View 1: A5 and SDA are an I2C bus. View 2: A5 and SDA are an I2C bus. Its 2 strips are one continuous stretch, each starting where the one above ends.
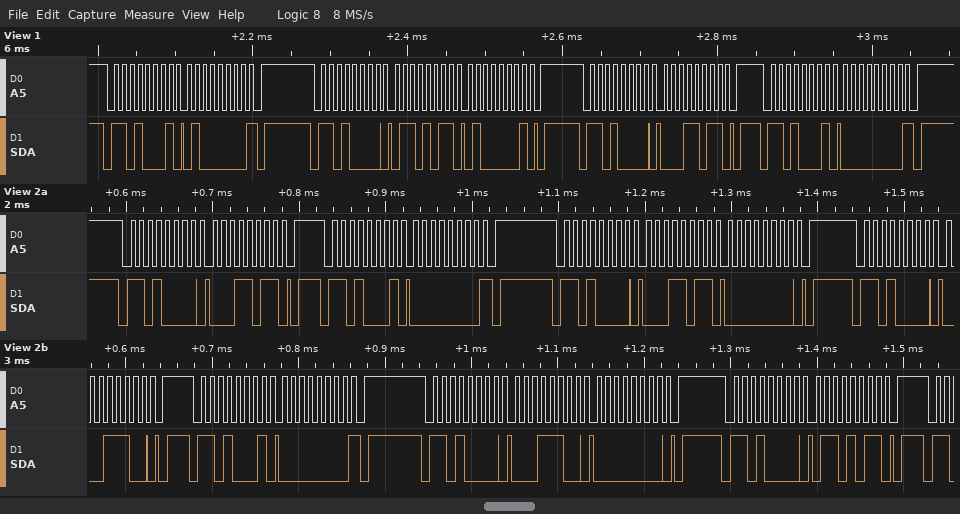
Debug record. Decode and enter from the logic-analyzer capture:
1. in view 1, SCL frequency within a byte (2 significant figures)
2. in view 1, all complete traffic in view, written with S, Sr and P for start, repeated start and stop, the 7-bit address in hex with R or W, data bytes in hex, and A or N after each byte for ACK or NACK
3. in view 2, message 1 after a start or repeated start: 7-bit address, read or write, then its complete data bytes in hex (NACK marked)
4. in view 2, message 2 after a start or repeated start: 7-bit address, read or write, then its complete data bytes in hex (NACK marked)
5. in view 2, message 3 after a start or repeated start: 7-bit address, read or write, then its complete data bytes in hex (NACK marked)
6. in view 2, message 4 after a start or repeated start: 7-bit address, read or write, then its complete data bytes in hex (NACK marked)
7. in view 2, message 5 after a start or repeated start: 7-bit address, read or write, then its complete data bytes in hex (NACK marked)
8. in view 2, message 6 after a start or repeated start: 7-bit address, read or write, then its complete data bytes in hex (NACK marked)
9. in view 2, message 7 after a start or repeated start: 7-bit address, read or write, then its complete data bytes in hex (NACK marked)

100 kHz
S 68R A 40 N P S 68W A 6B A 41 A P S 68W A 1B A P S 68R A 00 N P
0x68 write: 1B
0x68 read: 00 NACK
0x68 write: 1B 00
0x68 write: 1C
0x68 read: 00 NACK
0x68 write: 1C 00
0x68 write: 6B
